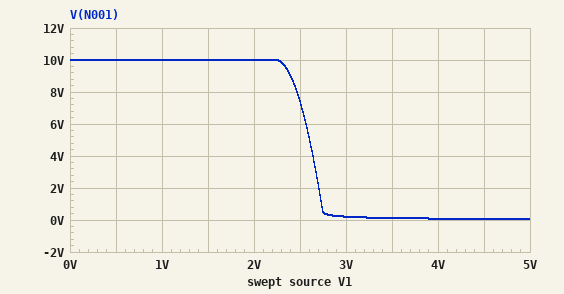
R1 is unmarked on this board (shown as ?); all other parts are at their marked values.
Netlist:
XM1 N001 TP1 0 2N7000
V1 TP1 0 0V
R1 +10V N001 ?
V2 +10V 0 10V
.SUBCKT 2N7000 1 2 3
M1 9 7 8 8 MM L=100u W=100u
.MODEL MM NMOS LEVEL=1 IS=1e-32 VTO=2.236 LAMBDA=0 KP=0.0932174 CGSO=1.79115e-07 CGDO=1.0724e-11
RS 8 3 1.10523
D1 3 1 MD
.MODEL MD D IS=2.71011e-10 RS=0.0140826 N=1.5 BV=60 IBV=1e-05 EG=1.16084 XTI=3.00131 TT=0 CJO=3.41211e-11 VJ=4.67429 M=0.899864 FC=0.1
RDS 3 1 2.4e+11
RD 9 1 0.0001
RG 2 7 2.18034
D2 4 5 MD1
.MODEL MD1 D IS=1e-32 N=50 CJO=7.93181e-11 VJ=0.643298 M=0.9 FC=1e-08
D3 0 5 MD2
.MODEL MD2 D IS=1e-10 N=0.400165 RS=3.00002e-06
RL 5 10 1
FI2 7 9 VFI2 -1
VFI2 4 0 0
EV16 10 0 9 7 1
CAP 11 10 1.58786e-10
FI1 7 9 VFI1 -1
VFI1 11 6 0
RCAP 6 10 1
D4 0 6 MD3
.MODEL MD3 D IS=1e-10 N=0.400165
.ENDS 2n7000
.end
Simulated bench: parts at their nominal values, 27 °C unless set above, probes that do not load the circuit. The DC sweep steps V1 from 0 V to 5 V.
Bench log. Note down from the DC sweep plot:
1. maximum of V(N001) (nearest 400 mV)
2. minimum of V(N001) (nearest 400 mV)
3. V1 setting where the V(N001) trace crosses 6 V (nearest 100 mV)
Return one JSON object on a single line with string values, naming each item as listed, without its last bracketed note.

{"maximum of V(N001)": "10.0 V", "minimum of V(N001)": "0 V", "V1 setting where the V(N001) trace crosses 6 V": "2.6 V"}
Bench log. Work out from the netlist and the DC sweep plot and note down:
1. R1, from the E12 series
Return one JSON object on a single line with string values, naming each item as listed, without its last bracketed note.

{"R1, from the E12 series": "820 Ω"}
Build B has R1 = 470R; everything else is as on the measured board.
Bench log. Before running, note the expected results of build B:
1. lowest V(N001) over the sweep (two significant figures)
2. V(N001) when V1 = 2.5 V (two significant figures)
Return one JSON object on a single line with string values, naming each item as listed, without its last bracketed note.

{"lowest V(N001) over the sweep": "110 mV", "V(N001) when V1 = 2.5 V": "8.5 V"}
